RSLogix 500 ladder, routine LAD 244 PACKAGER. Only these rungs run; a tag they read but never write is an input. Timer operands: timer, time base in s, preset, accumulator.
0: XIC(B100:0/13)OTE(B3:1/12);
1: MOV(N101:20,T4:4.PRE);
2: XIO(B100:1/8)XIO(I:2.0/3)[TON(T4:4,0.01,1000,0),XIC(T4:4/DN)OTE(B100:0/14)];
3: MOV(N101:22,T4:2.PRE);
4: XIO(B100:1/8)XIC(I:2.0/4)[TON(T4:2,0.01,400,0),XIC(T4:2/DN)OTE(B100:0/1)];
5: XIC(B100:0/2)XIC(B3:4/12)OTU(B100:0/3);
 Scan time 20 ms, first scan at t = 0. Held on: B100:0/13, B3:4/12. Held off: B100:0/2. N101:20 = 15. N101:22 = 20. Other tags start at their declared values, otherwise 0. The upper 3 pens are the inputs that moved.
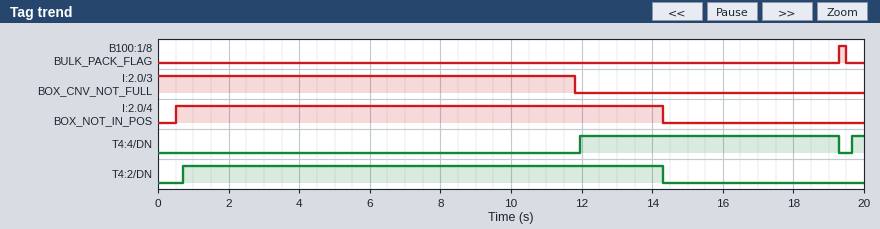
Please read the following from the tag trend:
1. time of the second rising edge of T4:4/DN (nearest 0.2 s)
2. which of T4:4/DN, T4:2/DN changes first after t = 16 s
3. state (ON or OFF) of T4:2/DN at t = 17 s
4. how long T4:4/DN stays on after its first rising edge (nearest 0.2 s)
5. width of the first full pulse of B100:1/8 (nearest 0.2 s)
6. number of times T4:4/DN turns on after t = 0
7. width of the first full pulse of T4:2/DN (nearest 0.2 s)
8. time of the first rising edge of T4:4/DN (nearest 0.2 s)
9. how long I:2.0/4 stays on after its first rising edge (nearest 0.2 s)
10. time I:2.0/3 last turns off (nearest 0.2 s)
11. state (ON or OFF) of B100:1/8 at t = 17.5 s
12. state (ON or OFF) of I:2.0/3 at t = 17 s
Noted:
19.6 s
T4:4/DN
OFF
7.4 s
0.2 s
2
13.6 s
12.0 s
13.8 s
11.8 s
OFF
OFF
